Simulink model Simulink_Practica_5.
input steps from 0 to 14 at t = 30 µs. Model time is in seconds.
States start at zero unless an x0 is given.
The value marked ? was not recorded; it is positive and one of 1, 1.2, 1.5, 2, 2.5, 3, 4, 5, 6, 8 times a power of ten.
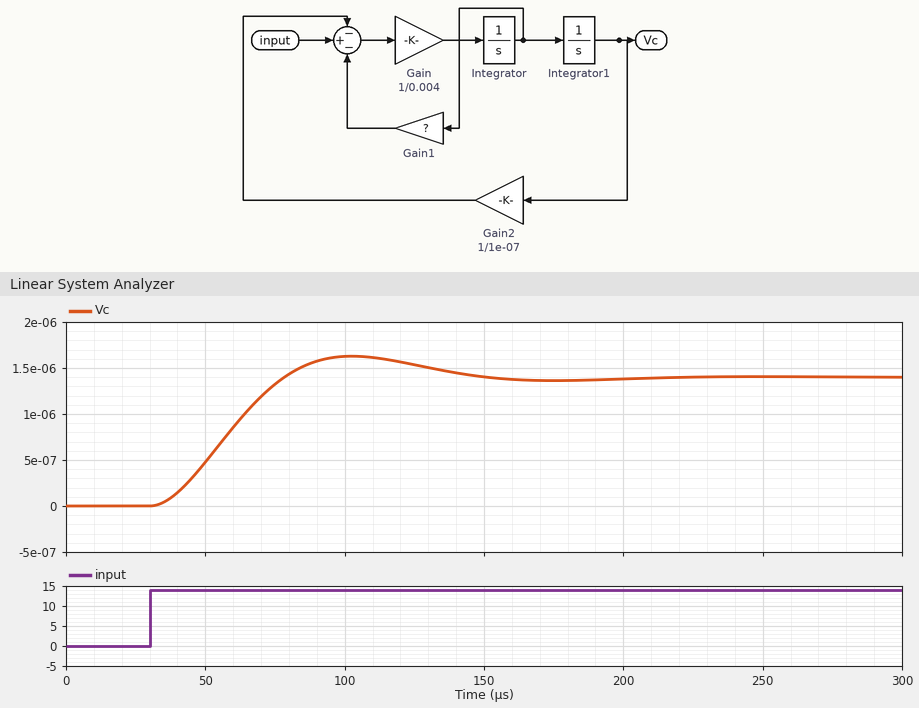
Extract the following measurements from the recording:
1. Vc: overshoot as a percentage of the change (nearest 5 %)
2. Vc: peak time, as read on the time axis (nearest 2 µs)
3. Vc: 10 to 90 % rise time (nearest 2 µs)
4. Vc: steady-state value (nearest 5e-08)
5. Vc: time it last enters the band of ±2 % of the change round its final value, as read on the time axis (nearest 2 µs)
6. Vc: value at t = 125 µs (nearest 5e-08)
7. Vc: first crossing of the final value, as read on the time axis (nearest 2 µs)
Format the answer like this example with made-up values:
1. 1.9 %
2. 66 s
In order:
1. 15 %
2. 102 µs
3. 32 µs
4. 0.00000140
5. 192 µs
6. 0.00000155
7. 78 µs
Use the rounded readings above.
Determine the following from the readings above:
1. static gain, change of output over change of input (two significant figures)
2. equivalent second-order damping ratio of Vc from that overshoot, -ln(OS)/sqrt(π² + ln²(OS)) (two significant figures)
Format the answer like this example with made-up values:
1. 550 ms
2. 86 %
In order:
1. 0.00000010
2. 0.52
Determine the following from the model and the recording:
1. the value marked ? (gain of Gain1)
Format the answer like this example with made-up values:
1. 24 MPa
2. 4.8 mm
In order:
1. 200
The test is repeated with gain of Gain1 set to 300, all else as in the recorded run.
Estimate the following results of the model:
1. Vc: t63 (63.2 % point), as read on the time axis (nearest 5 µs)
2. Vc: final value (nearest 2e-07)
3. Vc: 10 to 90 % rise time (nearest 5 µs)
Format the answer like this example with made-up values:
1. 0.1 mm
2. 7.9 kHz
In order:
1. 65 µs
2. 0.0000014
3. 45 µs
